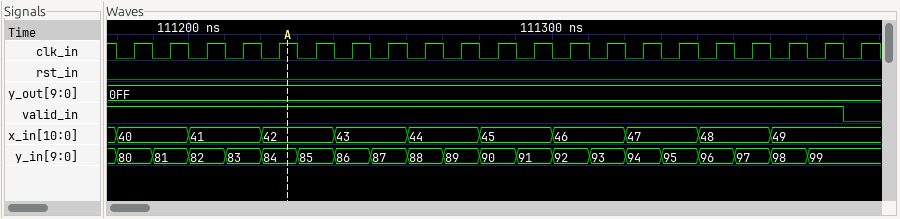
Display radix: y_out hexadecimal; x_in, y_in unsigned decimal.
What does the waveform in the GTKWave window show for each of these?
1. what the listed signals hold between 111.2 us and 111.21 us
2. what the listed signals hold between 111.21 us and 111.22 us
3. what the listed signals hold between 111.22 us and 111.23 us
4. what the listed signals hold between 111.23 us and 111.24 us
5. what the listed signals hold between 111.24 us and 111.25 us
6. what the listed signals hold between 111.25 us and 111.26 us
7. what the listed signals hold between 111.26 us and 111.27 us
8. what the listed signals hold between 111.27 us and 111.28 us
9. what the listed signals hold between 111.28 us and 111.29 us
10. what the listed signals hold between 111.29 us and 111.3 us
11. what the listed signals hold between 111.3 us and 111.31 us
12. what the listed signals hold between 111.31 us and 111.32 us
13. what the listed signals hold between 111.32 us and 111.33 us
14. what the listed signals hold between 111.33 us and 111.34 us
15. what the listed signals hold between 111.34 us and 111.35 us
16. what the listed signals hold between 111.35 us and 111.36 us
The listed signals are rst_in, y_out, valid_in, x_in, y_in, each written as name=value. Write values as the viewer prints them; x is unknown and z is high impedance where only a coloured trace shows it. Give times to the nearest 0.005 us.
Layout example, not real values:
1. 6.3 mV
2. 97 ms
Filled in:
1. rst_in=0, y_out=0FF, valid_in=1, x_in=41, y_in=82
2. rst_in=0, y_out=0FF, valid_in=1, x_in=41, y_in=83
3. rst_in=0, y_out=0FF, valid_in=1, x_in=42, y_in=84
4. rst_in=0, y_out=0FF, valid_in=1, x_in=42, y_in=85
5. rst_in=0, y_out=0FF, valid_in=1, x_in=43, y_in=86
6. rst_in=0, y_out=0FF, valid_in=1, x_in=43, y_in=87
7. rst_in=0, y_out=0FF, valid_in=1, x_in=44, y_in=88
8. rst_in=0, y_out=0FF, valid_in=1, x_in=44, y_in=89
9. rst_in=0, y_out=0FF, valid_in=1, x_in=45, y_in=90
10. rst_in=0, y_out=0FF, valid_in=1, x_in=45, y_in=91
11. rst_in=0, y_out=0FF, valid_in=1, x_in=46, y_in=92
12. rst_in=0, y_out=0FF, valid_in=1, x_in=46, y_in=93
13. rst_in=0, y_out=0FF, valid_in=1, x_in=47, y_in=94
14. rst_in=0, y_out=0FF, valid_in=1, x_in=47, y_in=95
15. rst_in=0, y_out=0FF, valid_in=1, x_in=48, y_in=96
16. rst_in=0, y_out=0FF, valid_in=1, x_in=48, y_in=97
